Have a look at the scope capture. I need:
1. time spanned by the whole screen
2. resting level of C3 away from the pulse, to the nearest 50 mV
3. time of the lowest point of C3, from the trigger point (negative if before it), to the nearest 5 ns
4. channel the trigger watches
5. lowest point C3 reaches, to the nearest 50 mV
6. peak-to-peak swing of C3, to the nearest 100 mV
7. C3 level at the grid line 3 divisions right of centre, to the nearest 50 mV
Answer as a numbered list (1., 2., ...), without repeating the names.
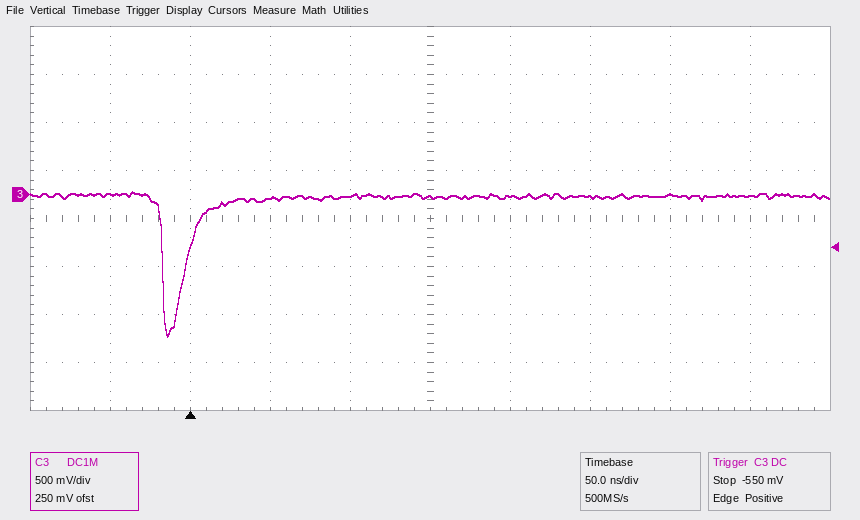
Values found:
1. 500 ns
2. 0 mV
3. -15 ns
4. C3
5. -1.50 V
6. 1.50 V
7. 0 mV
